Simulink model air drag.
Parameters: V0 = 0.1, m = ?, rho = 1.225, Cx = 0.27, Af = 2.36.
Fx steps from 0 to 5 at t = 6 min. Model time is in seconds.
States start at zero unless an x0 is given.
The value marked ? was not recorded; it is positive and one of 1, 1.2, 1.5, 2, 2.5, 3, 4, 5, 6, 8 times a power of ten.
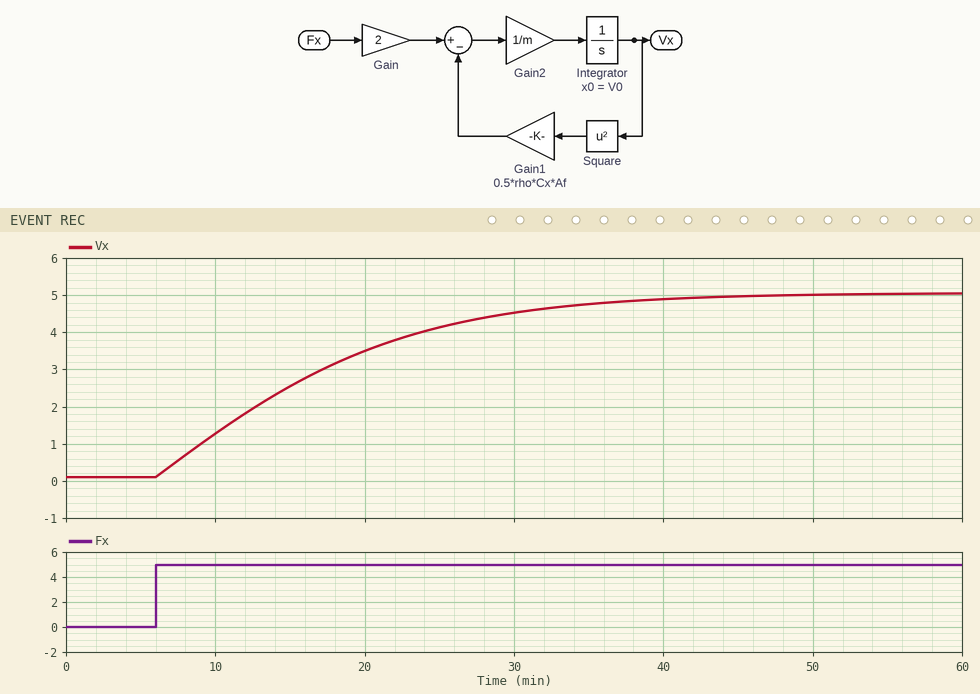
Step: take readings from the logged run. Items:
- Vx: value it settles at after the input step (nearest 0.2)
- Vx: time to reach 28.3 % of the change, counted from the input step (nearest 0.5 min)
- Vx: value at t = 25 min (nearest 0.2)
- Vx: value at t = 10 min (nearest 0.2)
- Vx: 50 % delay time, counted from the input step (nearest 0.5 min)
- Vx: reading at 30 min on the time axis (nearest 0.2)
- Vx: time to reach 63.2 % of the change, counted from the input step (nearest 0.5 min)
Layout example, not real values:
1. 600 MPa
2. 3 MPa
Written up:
1. 5.0
2. 5.0 min
3. 4.2
4. 1.2
5. 9.0 min
6. 4.6
7. 12.5 min
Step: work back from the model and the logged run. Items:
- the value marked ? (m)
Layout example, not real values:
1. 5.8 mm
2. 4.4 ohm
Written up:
1. 2000
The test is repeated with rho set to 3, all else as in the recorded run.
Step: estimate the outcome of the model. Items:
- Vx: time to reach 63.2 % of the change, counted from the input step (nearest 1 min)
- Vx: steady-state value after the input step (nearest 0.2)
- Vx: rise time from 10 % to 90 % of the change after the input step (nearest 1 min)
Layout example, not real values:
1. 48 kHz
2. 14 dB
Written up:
1. 8 min
2. 3.2
3. 15 min
